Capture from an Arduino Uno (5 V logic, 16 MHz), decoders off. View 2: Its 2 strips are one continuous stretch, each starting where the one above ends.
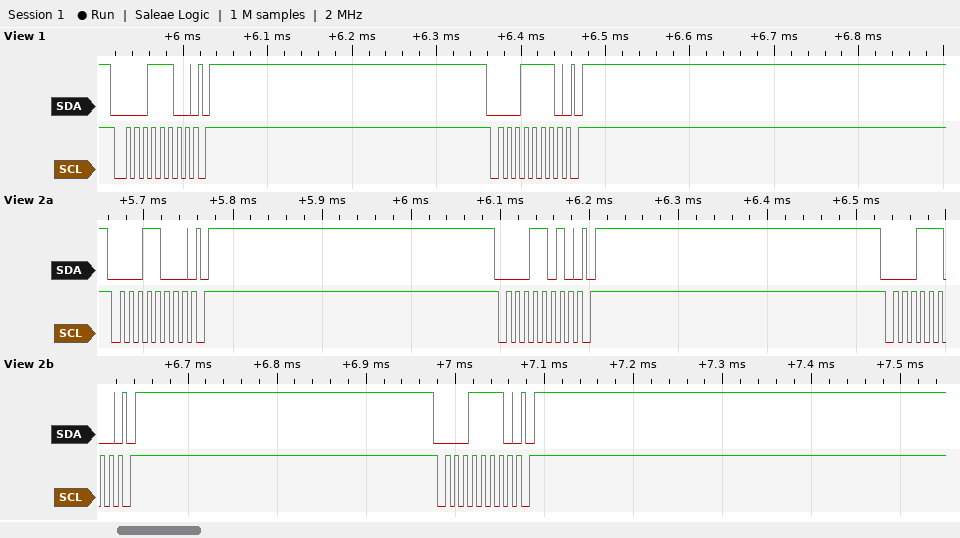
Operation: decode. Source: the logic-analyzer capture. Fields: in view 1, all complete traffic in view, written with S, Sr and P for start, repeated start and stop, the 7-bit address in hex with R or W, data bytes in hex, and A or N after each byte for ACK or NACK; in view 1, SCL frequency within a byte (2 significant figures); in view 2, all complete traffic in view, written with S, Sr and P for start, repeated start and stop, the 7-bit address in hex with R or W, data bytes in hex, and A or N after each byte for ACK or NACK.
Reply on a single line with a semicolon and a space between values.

S 0EW A P S 0FW A P; 100 kHz; S 0CW A P S 0DW A P S 0EW A P S 0FW A P
